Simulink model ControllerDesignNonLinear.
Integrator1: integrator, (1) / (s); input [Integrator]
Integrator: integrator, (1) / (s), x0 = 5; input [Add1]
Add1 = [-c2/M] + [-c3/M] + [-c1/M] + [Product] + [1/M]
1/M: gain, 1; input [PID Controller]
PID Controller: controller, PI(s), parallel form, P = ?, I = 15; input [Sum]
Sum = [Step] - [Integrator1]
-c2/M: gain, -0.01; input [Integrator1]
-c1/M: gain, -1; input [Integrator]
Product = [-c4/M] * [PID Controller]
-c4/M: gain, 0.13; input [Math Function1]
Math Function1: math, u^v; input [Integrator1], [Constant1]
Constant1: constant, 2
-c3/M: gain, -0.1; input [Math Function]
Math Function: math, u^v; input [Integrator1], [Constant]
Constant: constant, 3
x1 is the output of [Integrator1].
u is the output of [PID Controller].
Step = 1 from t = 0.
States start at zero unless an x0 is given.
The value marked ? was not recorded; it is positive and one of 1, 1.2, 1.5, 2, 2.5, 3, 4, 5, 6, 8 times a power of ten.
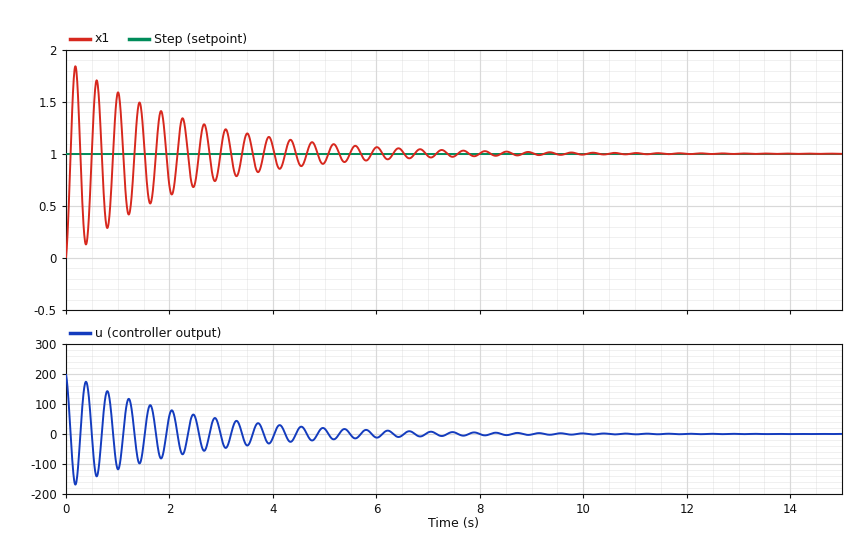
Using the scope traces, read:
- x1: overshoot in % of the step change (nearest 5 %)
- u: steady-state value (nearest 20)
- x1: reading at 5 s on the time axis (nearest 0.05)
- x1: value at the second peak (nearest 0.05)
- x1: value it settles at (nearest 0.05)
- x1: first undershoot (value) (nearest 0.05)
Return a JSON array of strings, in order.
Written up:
["85 %", "0", "0.90", "1.70", "1.00", "0.15"]
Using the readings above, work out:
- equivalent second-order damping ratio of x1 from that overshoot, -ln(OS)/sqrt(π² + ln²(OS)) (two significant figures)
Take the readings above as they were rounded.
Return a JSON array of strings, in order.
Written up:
["0.052"]
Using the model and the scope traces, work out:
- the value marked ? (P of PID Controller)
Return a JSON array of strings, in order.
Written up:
["200"]
